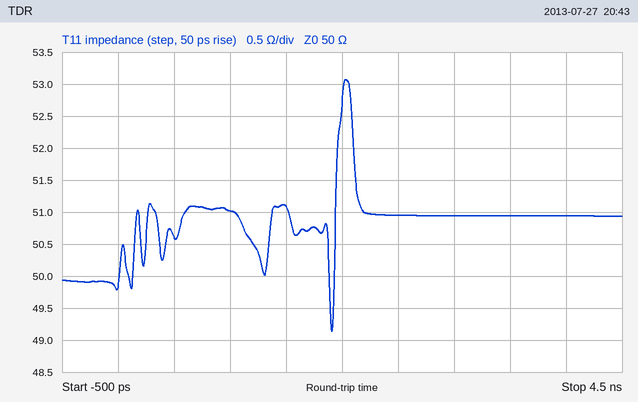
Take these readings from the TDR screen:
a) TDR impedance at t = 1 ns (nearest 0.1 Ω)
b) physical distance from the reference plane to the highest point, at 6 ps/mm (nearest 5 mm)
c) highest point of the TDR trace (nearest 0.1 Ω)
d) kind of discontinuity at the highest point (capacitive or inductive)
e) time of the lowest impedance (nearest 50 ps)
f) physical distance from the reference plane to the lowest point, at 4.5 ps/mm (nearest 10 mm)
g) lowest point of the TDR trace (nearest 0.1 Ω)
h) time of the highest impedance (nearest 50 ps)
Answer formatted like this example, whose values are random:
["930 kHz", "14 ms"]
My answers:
["51.0 Ω", "170 mm", "53.1 Ω", "inductive", "1.90 ns", "210 mm", "49.1 Ω", "2.05 ns"]
